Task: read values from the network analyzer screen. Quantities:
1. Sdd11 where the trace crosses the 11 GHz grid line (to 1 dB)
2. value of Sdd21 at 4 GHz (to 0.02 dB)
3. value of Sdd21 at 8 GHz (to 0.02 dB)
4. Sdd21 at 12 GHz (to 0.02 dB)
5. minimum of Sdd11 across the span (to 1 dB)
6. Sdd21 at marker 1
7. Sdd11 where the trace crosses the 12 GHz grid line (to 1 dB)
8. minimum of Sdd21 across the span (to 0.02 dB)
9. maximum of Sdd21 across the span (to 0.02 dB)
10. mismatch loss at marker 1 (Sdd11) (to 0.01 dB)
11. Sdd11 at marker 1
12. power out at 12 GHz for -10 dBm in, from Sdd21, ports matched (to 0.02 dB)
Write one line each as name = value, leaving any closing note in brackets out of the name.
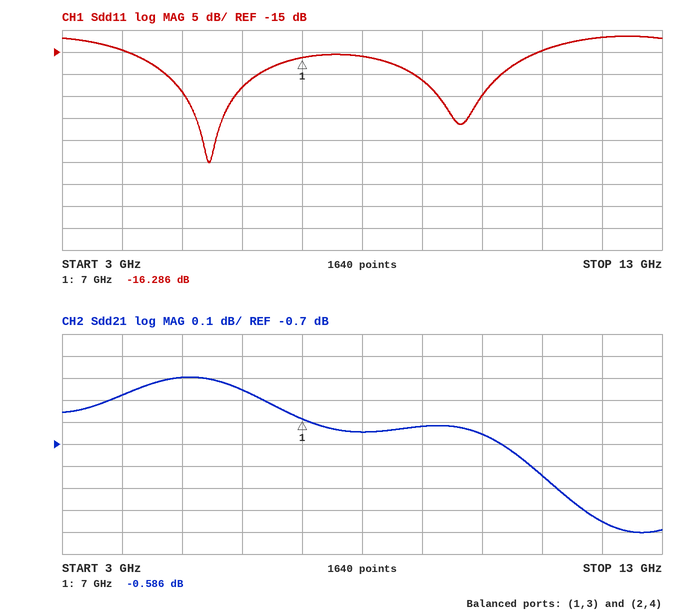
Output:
Sdd11 where the trace crosses the 11 GHz grid line = -15 dB
value of Sdd21 at 4 GHz = -0.48 dB
value of Sdd21 at 8 GHz = -0.64 dB
Sdd21 at 12 GHz = -1.06 dB
minimum of Sdd11 across the span = -40 dB
Sdd21 at marker 1 = -0.586 dB
Sdd11 where the trace crosses the 12 GHz grid line = -12 dB
minimum of Sdd21 across the span = -1.10 dB
maximum of Sdd21 across the span = -0.40 dB
mismatch loss at marker 1 (Sdd11) = 0.10 dB
Sdd11 at marker 1 = -16.286 dB
power out at 12 GHz for -10 dBm in, from Sdd21, ports matched = -11.06 dBm
